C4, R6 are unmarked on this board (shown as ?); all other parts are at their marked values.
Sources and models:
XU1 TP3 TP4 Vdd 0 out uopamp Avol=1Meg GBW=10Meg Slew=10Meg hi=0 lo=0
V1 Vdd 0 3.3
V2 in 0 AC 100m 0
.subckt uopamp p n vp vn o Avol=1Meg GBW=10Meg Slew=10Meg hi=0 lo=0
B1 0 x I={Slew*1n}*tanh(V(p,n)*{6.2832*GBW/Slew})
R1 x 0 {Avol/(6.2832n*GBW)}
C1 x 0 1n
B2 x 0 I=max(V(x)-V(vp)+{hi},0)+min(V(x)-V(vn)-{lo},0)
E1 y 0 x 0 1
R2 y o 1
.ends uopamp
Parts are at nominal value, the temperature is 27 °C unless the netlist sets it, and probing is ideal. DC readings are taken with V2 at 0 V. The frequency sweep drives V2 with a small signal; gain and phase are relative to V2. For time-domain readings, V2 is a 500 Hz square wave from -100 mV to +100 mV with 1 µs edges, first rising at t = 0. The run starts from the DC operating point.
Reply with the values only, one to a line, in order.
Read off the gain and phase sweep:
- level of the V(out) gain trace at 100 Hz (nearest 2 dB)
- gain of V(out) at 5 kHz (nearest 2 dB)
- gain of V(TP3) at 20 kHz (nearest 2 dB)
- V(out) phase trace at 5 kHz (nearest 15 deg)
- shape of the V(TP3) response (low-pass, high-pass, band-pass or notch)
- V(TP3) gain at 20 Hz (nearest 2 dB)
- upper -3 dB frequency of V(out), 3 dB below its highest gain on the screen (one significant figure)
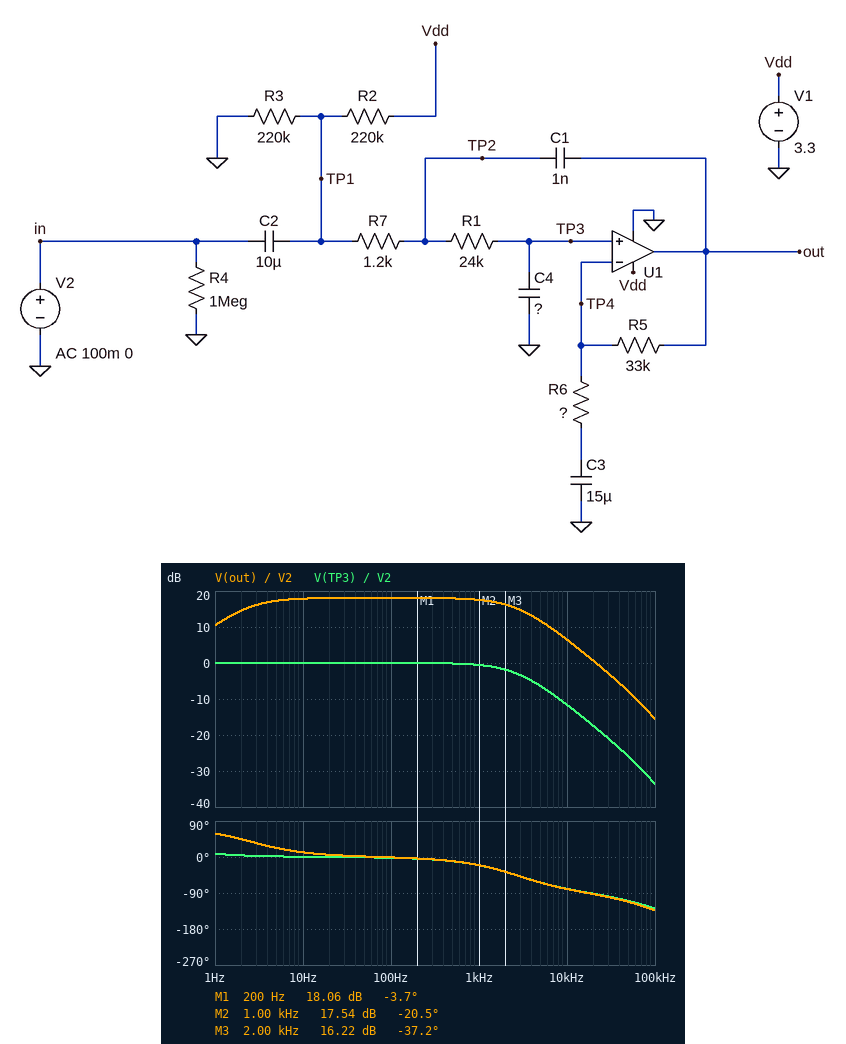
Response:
18 dB
12 dB
-18 dB
-60 deg
low-pass
0 dB
3 kHz
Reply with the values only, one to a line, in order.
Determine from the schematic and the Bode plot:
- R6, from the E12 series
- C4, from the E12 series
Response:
4.7 kΩ
2.7 nF
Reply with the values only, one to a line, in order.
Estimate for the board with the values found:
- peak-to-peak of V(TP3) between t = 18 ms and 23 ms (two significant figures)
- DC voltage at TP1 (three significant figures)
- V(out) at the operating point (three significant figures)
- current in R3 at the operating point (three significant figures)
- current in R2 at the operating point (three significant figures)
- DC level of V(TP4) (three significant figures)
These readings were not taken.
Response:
200 mV
1.65 V
1.65 V
7.50 µA
7.50 µA
1.65 V
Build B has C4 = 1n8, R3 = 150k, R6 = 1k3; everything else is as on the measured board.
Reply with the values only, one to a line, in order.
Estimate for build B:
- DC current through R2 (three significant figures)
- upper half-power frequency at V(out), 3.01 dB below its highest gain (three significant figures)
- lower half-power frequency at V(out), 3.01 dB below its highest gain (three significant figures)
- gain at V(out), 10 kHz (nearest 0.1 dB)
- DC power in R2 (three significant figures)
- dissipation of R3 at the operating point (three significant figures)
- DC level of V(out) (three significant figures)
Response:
8.92 µA
14.1 kHz
8.15 Hz
26.9 dB
17.5 µW
11.9 µW
1.34 V
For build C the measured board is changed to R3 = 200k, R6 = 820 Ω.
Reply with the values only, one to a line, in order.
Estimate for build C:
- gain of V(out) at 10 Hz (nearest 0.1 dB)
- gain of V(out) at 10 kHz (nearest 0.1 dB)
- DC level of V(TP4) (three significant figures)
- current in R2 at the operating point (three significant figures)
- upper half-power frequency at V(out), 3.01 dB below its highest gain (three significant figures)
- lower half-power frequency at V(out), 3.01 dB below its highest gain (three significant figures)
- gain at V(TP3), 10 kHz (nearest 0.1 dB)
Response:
28.0 dB
29.6 dB
1.57 V
7.86 µA
10.6 kHz
12.9 Hz
-2.7 dB
